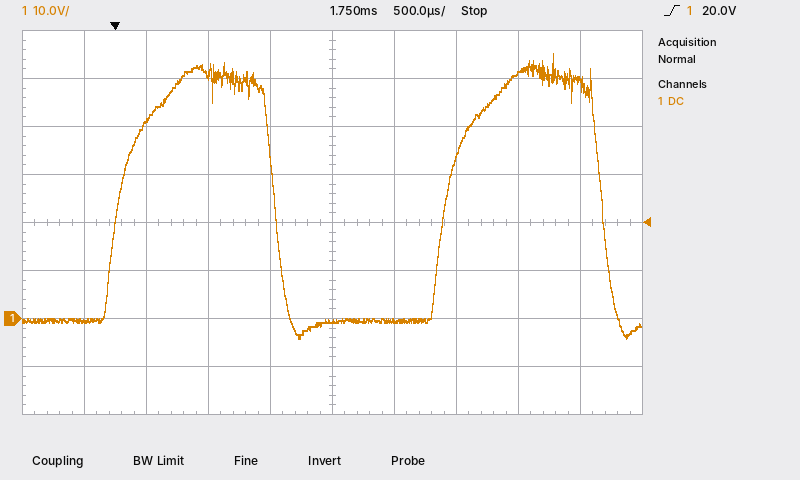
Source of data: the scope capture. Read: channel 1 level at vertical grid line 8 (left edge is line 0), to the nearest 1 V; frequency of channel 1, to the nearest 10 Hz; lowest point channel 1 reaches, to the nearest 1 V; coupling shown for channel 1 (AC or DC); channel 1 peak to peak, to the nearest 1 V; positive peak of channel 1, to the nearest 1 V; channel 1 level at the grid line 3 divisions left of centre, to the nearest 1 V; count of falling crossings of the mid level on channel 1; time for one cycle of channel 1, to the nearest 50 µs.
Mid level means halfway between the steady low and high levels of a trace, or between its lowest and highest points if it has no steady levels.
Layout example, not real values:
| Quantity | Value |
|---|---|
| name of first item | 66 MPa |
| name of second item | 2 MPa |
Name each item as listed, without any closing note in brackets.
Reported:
| Quantity | Value |
|---|---|
| channel 1 level at vertical grid line 8 (left edge is line 0), to the nearest 1 V | 51 V |
| frequency of channel 1, to the nearest 10 Hz | 380 Hz |
| lowest point channel 1 reaches, to the nearest 1 V | -4 V |
| coupling shown for channel 1 | DC |
| channel 1 peak to peak, to the nearest 1 V | 59 V |
| positive peak of channel 1, to the nearest 1 V | 55 V |
| channel 1 level at the grid line 3 divisions left of centre, to the nearest 1 V | 41 V |
| count of falling crossings of the mid level on channel 1 | 2 |
| time for one cycle of channel 1, to the nearest 50 µs | 2.65 ms |
